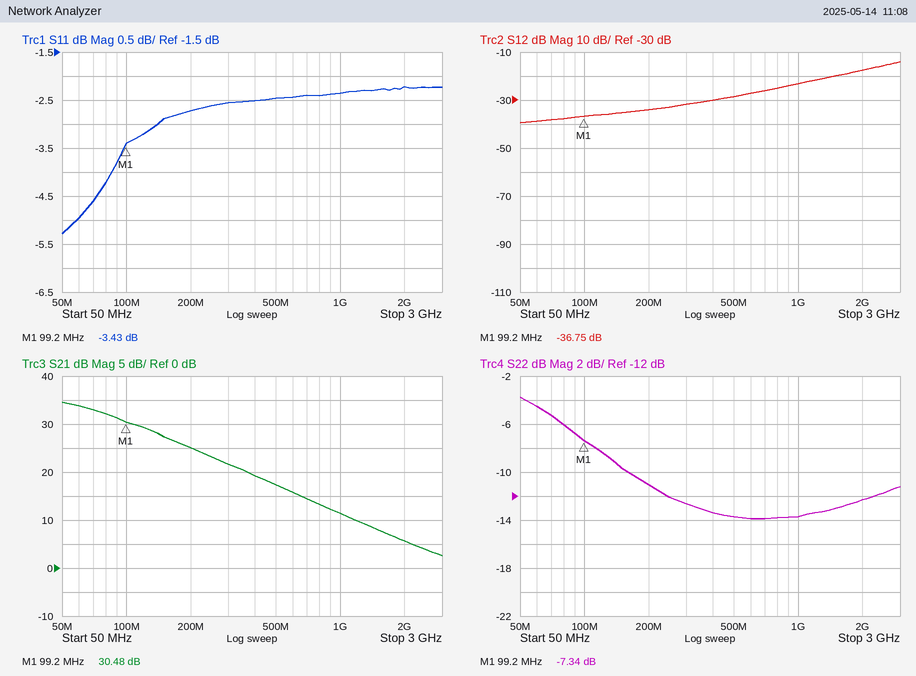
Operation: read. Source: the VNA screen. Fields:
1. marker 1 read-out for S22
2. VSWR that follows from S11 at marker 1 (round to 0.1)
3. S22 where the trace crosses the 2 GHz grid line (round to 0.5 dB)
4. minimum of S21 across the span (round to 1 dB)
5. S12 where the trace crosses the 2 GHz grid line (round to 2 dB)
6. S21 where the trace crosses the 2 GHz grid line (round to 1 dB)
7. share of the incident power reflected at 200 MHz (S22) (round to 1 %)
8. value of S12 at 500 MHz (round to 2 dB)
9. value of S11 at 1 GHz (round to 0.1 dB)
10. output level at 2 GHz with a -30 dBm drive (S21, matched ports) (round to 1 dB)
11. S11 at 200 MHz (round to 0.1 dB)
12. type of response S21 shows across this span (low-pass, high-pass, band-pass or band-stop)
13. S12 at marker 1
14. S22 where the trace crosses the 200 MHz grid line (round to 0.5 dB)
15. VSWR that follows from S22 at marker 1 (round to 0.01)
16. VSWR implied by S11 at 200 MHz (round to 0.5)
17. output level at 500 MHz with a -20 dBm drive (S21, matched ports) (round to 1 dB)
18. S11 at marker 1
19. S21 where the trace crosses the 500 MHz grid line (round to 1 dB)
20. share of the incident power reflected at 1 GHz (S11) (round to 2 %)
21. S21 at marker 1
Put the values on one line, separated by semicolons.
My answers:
-7.34 dB; 5.1; -12.5 dB; 3 dB; -18 dB; 6 dB; 8 %; -28 dB; -2.4 dB; -24 dBm; -2.7 dB; low-pass; -36.75 dB; -11.0 dB; 2.51; 6.5; -3 dBm; -3.43 dB; 17 dB; 58 %; 30.48 dB
